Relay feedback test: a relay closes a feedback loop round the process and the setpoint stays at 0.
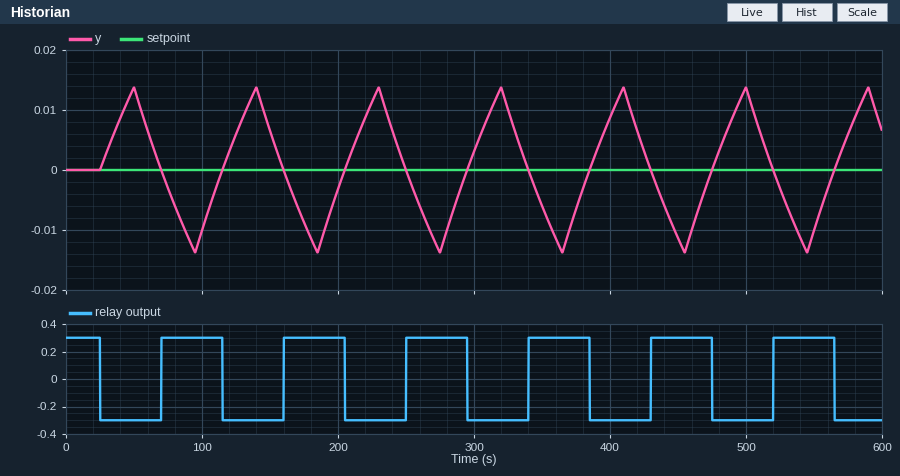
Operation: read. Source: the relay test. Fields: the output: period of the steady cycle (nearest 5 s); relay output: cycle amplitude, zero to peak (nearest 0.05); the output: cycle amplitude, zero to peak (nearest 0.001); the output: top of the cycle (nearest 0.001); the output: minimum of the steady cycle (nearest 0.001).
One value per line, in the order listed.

90 s
0.30
0.014
0.014
-0.014
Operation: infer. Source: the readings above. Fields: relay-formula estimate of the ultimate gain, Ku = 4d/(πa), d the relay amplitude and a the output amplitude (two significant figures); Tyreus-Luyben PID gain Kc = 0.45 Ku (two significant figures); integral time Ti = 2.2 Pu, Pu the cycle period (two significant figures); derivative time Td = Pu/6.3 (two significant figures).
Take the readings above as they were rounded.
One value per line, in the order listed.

27
12
200 s
14 s
